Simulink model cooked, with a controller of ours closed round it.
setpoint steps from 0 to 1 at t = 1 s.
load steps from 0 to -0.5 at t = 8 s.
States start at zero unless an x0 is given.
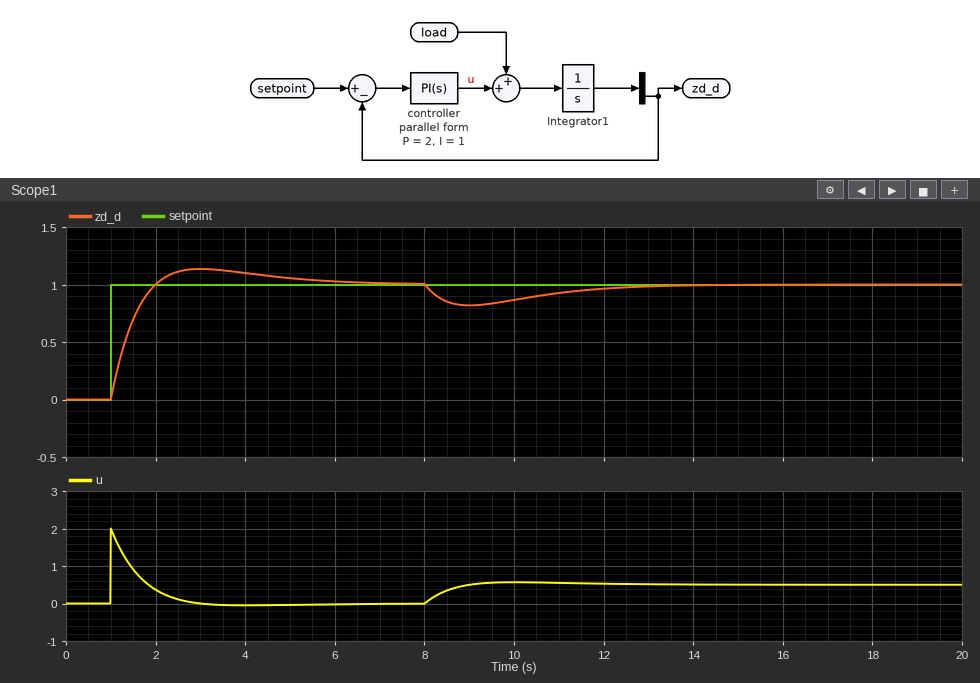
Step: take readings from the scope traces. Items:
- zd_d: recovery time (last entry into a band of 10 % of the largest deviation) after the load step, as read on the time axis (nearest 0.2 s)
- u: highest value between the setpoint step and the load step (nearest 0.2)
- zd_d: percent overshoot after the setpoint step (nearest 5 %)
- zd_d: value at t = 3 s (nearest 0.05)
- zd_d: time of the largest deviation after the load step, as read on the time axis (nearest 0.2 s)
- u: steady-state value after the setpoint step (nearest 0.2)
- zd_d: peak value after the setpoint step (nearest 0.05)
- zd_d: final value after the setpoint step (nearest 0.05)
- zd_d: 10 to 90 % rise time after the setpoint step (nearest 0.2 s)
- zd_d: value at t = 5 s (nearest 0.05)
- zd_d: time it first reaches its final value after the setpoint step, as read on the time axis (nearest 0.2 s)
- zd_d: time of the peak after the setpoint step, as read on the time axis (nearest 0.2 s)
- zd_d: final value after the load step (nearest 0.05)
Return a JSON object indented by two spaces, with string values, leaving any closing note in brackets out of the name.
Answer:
{
  "zd_d: recovery time (last entry into a band of 10 % of the largest deviation) after the load step, as read on the time axis": "12.8 s",
  "u: highest value between the setpoint step and the load step": "2.0",
  "zd_d: percent overshoot after the setpoint step": "15 %",
  "zd_d: value at t = 3 s": "1.15",
  "zd_d: time of the largest deviation after the load step, as read on the time axis": "9.0 s",
  "u: steady-state value after the setpoint step": "0.0",
  "zd_d: peak value after the setpoint step": "1.15",
  "zd_d: final value after the setpoint step": "1.00",
  "zd_d: 10 to 90 % rise time after the setpoint step": "0.8 s",
  "zd_d: value at t = 5 s": "1.05",
  "zd_d: time it first reaches its final value after the setpoint step, as read on the time axis": "2.0 s",
  "zd_d: time of the peak after the setpoint step, as read on the time axis": "3.0 s",
  "zd_d: final value after the load step": "1.00"
}
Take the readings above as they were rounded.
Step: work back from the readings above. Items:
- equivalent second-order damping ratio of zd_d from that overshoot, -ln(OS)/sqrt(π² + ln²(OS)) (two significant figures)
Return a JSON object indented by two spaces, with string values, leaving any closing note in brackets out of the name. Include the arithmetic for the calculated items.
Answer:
{
  "equivalent second-order damping ratio of zd_d from that overshoot, -ln(OS)/sqrt(π² + ln²(OS))": "ln(0.15) = -1.897; 1.897 / sqrt(9.870 + 3.599) = 0.52"
}
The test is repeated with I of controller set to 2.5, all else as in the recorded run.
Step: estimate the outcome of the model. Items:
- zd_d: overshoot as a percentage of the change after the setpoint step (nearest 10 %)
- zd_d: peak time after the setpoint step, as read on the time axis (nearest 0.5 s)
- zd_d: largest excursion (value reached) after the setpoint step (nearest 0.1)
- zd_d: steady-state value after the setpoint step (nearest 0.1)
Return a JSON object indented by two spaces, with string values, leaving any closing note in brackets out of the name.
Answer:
{
  "zd_d: overshoot as a percentage of the change after the setpoint step": "20 %",
  "zd_d: peak time after the setpoint step, as read on the time axis": "2.5 s",
  "zd_d: largest excursion (value reached) after the setpoint step": "1.2",
  "zd_d: steady-state value after the setpoint step": "1.0"
}
